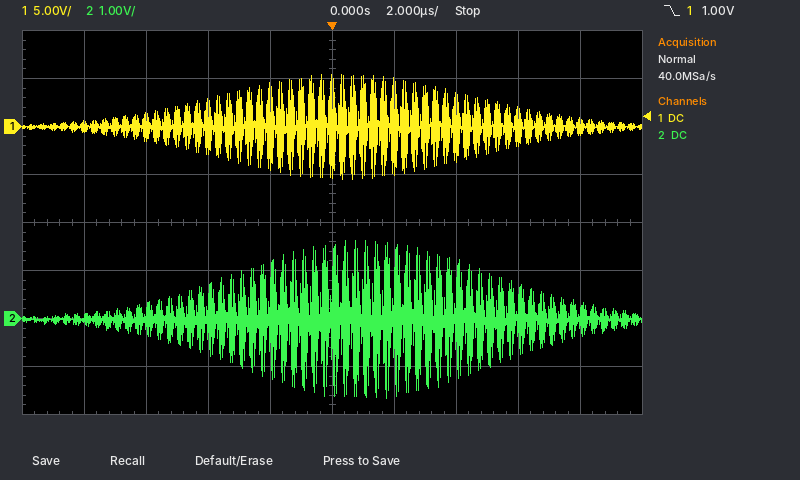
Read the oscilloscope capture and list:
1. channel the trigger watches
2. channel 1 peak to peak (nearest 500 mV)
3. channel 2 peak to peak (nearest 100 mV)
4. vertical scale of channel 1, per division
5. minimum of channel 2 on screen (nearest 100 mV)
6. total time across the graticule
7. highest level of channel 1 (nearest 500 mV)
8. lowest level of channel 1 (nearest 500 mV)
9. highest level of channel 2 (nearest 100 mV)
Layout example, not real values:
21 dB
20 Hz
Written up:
channel 1
11.0 V
3.3 V
5 V
-1.7 V
20 µs
5.5 V
-5.5 V
1.6 V
